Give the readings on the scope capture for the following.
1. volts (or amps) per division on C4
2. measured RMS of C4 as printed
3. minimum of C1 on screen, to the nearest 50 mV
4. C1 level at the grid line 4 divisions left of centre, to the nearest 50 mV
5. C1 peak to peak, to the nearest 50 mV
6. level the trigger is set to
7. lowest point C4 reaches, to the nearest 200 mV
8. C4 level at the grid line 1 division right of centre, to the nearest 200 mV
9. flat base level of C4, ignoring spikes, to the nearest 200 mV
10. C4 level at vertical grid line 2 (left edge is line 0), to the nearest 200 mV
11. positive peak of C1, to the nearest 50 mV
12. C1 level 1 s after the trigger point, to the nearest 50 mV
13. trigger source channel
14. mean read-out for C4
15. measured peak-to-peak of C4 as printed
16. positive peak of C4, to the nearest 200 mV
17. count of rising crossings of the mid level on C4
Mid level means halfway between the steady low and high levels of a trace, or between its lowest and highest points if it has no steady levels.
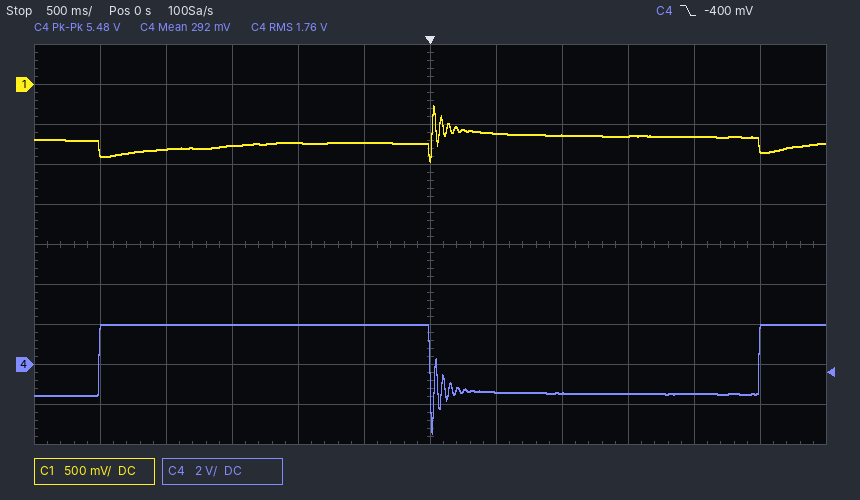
2 V
1.76 V
-950 mV
-800 mV
700 mV
-400 mV
-3.4 V
-1.4 V
-1.4 V
2.0 V
-250 mV
-650 mV
C4
292 mV
5.48 V
2.0 V
2
